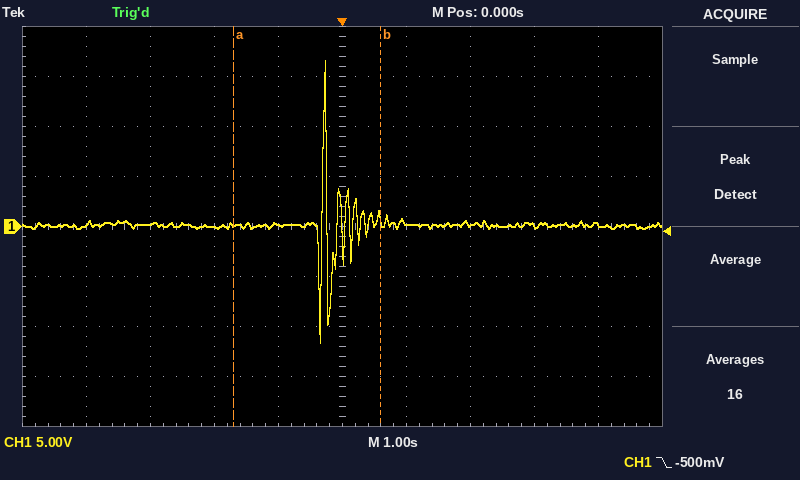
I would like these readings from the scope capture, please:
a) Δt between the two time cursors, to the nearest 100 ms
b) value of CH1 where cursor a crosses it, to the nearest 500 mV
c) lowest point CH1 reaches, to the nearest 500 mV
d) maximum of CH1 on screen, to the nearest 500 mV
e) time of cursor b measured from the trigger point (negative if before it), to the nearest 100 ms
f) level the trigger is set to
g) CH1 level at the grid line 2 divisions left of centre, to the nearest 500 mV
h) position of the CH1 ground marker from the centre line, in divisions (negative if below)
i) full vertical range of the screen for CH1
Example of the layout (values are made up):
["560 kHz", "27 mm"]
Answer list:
["2.3 s", "0.0 V", "-11.5 V", "16.5 V", "+600 ms", "-500 mV", "0.0 V", "0.0 div", "40 V"]
